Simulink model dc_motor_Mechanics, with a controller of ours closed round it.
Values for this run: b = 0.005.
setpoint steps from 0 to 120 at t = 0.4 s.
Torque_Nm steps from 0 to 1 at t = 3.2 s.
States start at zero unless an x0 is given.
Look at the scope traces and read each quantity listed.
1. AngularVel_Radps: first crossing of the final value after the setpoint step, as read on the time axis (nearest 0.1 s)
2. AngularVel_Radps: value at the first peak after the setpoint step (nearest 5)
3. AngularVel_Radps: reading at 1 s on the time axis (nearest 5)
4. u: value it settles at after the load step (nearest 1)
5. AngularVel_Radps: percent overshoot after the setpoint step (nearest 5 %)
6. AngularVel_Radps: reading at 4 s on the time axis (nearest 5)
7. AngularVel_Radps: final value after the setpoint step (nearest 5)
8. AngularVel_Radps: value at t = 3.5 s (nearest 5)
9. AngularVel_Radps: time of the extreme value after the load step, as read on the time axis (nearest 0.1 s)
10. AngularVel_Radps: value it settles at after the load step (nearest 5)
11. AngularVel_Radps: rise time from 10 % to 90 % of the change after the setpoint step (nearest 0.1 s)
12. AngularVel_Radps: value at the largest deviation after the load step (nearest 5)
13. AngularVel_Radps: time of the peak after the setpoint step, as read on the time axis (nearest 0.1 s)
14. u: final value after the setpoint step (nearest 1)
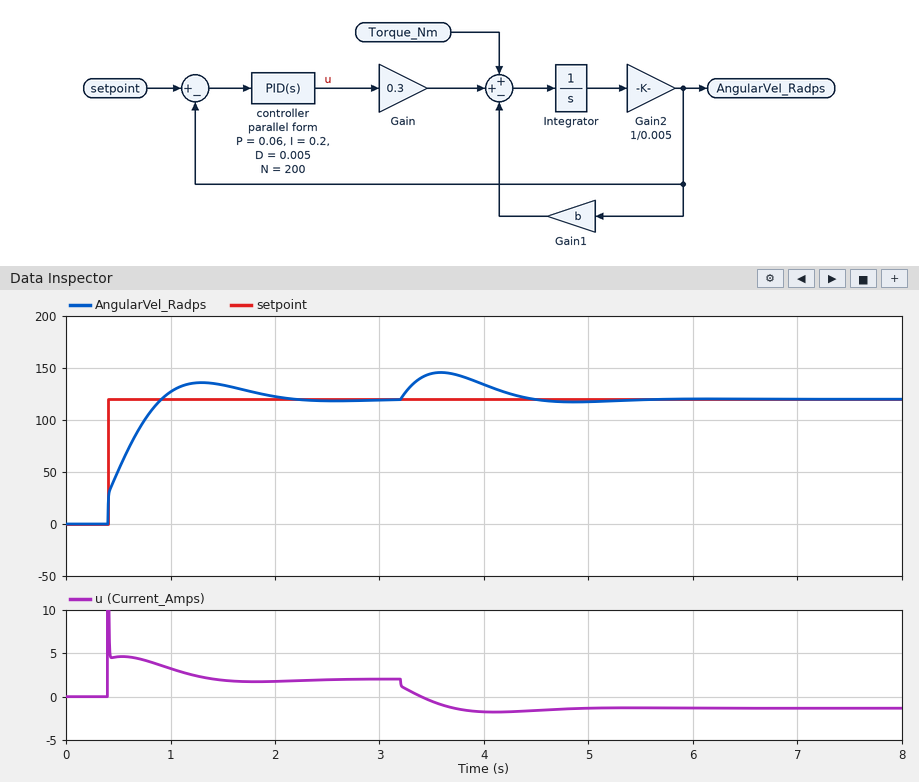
0.9 s
135
125
-1
15 %
135
120
145
3.6 s
120
0.4 s
145
1.3 s
2
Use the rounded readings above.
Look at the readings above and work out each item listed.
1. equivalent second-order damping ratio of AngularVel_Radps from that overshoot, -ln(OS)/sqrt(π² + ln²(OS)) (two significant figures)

0.52
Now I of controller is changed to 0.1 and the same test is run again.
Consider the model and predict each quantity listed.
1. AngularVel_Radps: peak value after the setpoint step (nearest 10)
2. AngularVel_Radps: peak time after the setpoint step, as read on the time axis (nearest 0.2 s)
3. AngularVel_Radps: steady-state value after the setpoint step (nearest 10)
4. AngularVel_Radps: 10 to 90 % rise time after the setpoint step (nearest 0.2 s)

130
1.8 s
120
0.6 s
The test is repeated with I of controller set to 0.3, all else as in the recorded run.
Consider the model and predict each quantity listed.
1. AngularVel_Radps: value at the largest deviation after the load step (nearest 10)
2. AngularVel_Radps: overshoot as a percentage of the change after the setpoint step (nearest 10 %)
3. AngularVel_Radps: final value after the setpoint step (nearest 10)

140
20 %
120
